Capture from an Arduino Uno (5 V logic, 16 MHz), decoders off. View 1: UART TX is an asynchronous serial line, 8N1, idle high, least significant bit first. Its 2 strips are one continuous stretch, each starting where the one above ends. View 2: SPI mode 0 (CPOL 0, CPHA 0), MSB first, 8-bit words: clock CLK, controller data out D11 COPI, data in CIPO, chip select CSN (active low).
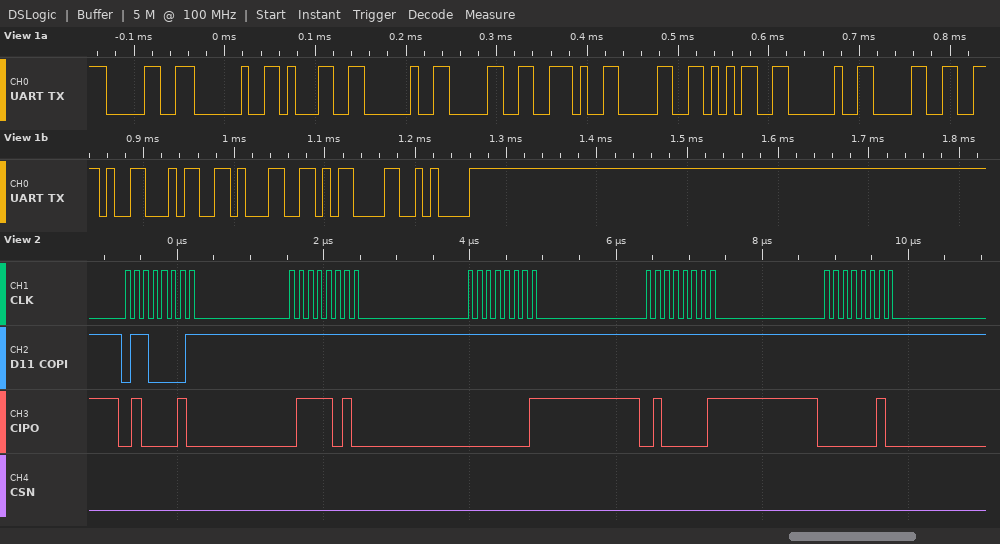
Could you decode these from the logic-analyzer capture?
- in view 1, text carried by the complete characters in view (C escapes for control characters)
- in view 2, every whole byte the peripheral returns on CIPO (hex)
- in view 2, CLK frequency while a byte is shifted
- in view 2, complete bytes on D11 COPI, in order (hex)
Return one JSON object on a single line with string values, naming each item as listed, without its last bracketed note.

{"in view 1, text carried by the complete characters in view": "\"0 1 0.05 0.41\\r\\n\"", "in view 2, every whole byte the peripheral returns on CIPO": "42 7A 01 41 02", "in view 2, CLK frequency while a byte is shifted": "8 MHz", "in view 2, complete bytes on D11 COPI, in order": "61 FF FF FF FF"}
